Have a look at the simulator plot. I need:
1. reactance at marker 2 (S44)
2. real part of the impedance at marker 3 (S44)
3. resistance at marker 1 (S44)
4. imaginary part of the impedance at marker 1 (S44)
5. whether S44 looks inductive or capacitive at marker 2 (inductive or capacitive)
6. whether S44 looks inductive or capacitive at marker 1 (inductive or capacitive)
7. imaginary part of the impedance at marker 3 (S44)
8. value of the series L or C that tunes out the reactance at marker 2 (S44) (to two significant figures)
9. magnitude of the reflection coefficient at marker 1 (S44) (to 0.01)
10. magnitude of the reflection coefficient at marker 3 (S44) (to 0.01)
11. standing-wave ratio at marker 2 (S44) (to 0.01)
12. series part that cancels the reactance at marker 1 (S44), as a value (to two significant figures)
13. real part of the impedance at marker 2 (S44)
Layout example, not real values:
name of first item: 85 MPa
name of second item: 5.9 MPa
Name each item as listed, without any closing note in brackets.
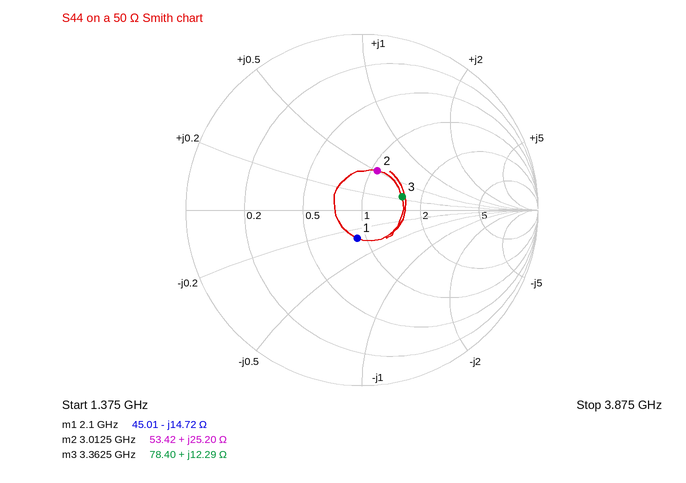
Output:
reactance at marker 2: +25.20 Ω
real part of the impedance at marker 3: 78.40 Ω
resistance at marker 1: 45.01 Ω
imaginary part of the impedance at marker 1: -14.72 Ω
whether S44 looks inductive or capacitive at marker 2: inductive
whether S44 looks inductive or capacitive at marker 1: capacitive
imaginary part of the impedance at marker 3: +12.29 Ω
value of the series L or C that tunes out the reactance at marker 2 (S44): 2.1 pF
magnitude of the reflection coefficient at marker 1 (S44): 0.16
magnitude of the reflection coefficient at marker 3 (S44): 0.24
standing-wave ratio at marker 2 (S44): 1.63
series part that cancels the reactance at marker 1 (S44), as a value: 1.1 nH
real part of the impedance at marker 2: 53.42 Ω
